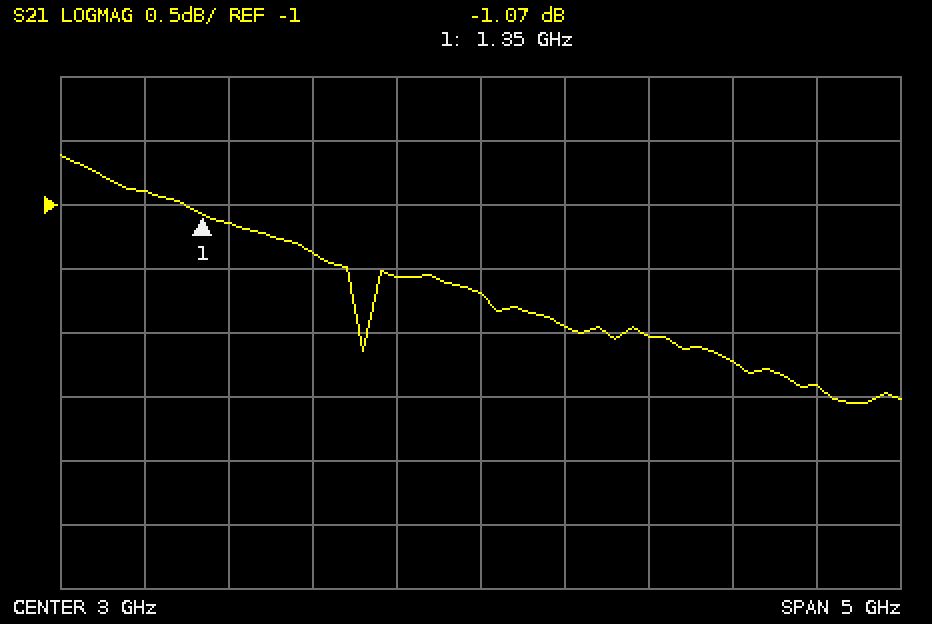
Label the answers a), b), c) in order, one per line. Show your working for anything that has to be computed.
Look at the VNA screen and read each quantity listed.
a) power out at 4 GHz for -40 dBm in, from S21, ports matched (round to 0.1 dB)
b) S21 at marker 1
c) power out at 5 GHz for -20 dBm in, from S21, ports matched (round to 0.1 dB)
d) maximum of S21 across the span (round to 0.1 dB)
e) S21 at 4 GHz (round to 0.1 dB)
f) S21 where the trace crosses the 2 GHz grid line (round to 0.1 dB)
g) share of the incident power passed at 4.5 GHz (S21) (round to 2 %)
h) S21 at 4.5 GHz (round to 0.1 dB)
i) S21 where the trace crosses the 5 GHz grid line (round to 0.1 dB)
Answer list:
a) -40 dBm + (-2.0 dB) = -42.0 dBm
b) -1.07 dB
c) -20 dBm + (-2.4 dB) = -22.4 dBm
d) -0.6 dB
e) -2.0 dB
f) -1.4 dB
g) 10^(-2.2/10) ≈ 60 %
h) -2.2 dB
i) -2.4 dB
